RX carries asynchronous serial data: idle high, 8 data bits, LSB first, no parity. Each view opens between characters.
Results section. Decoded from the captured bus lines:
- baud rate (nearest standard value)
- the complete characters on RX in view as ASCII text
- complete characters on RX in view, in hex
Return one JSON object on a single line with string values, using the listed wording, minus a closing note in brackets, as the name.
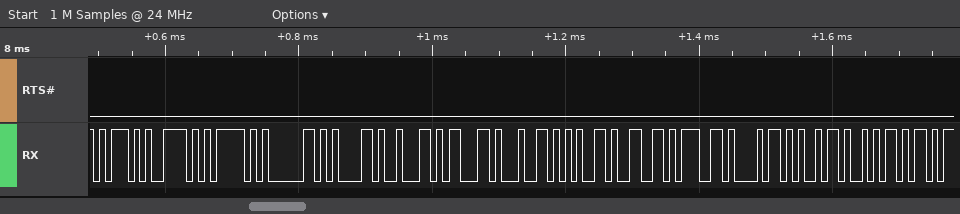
{"baud rate": "115200 baud", "the complete characters on RX in view as ASCII text": "\"]^_`abcdefghij\"", "complete characters on RX in view, in hex": "5D, 5E, 5F, 60, 61, 62, 63, 64, 65, 66, 67, 68, 69, 6A"}
